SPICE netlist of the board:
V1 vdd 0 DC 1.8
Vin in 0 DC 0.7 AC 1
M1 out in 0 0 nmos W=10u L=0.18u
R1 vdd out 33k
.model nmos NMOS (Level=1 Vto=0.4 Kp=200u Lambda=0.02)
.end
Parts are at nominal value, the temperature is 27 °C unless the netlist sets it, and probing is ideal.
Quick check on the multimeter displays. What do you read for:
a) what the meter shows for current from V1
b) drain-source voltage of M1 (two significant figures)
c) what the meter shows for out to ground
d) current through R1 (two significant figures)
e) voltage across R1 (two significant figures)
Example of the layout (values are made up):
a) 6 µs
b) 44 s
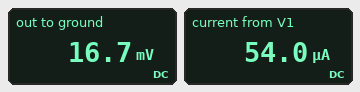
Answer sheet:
a) 54.0 µA
b) 17 mV
c) 16.7 mV
d) 54 µA
e) 1.8 V
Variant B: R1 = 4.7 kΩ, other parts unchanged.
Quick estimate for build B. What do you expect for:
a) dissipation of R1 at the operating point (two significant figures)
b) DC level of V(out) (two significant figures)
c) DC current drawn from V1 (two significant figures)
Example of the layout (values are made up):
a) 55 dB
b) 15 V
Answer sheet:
a) 590 µW
b) 140 mV
c) 350 µA
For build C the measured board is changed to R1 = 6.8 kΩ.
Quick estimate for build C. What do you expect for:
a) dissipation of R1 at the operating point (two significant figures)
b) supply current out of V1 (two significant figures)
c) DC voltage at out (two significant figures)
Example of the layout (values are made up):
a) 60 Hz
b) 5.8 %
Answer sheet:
a) 430 µW
b) 250 µA
c) 88 mV
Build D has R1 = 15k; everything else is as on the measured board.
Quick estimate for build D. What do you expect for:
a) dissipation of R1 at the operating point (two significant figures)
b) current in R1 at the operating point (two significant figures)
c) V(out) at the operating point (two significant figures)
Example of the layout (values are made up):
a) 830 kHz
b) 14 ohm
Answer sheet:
a) 210 µW
b) 120 µA
c) 38 mV
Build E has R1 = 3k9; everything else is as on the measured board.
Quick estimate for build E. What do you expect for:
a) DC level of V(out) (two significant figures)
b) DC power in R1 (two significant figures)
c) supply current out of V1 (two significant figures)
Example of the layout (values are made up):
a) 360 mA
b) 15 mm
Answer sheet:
a) 180 mV
b) 680 µW
c) 420 µA
